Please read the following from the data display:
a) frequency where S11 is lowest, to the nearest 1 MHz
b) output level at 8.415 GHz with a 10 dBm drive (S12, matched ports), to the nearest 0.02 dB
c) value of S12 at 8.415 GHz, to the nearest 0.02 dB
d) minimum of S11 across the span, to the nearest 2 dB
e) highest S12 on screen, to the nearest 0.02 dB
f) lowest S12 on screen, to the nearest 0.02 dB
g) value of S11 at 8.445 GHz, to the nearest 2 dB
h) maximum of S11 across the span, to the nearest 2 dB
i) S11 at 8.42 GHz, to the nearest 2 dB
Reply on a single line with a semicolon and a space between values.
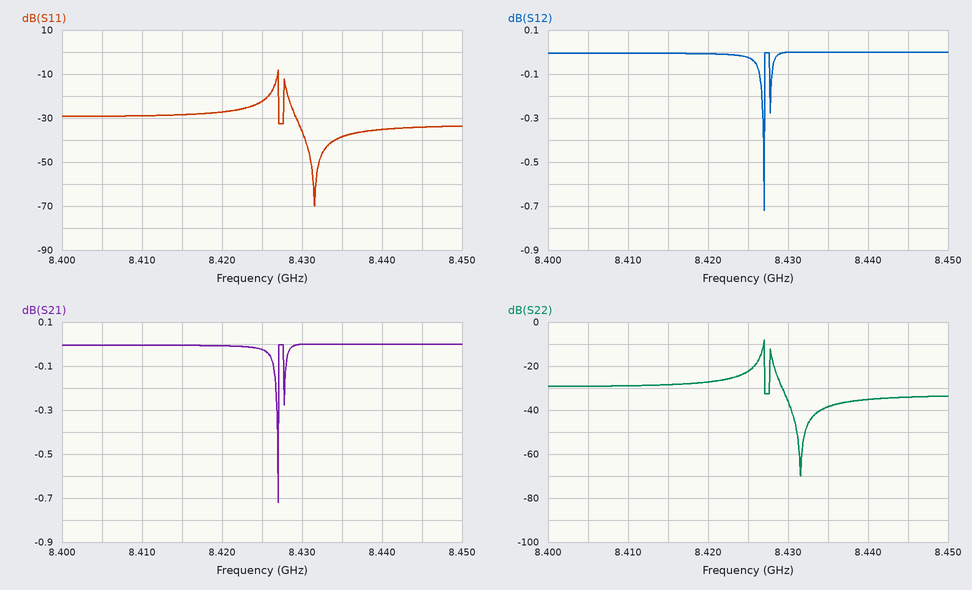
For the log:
8.432 GHz; 10.00 dBm; 0.00 dB; -70 dB; 0.00 dB; -0.72 dB; -34 dB; -8 dB; -28 dB
